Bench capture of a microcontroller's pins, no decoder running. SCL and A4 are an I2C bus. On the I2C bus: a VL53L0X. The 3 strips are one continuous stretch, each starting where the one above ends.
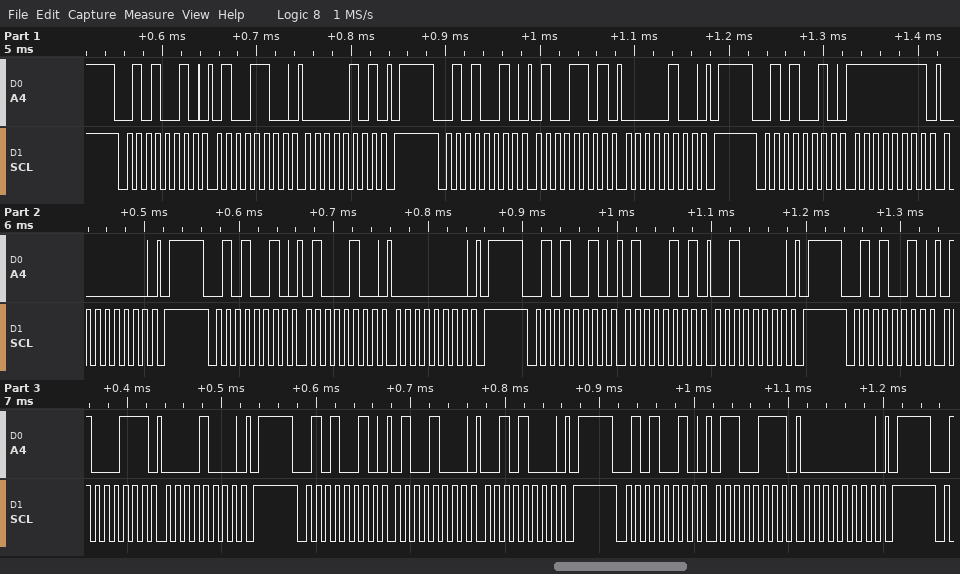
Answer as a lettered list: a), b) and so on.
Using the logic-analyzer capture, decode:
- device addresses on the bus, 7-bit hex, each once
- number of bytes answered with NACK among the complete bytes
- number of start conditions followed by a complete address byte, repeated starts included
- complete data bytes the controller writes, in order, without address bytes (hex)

a) 0x29
b) 0
c) 8
d) 4C 05 4D 04 FF 00 44 00 45 20 47 08 48 28 67 00
